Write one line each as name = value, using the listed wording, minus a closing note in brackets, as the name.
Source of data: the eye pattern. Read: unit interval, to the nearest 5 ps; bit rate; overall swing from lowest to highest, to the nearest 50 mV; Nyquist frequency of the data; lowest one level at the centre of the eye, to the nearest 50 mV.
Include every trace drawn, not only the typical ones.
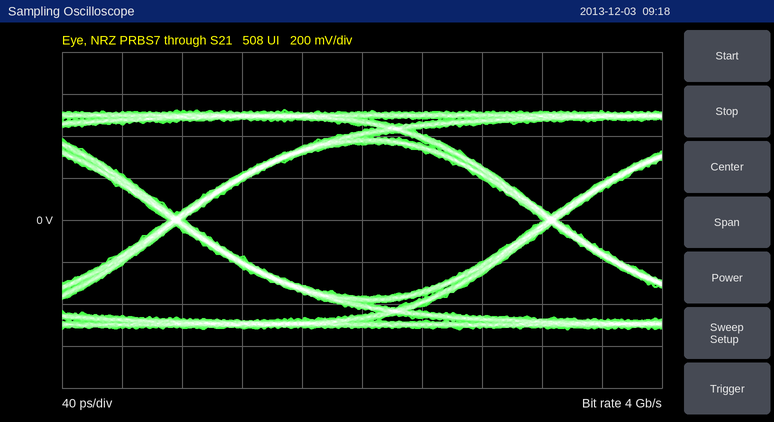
unit interval, to the nearest 5 ps = 250 ps
bit rate = 4 Gb/s
overall swing from lowest to highest, to the nearest 50 mV = 1.05 V
Nyquist frequency of the data = 2 GHz
lowest one level at the centre of the eye, to the nearest 50 mV = 350 mV
